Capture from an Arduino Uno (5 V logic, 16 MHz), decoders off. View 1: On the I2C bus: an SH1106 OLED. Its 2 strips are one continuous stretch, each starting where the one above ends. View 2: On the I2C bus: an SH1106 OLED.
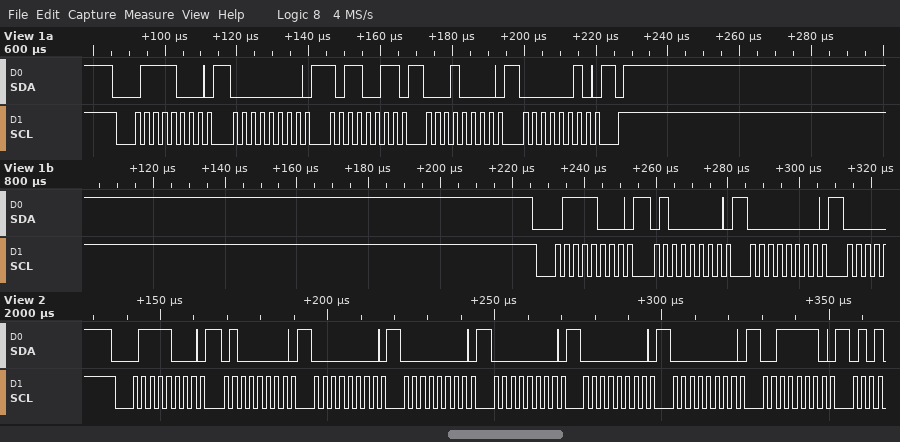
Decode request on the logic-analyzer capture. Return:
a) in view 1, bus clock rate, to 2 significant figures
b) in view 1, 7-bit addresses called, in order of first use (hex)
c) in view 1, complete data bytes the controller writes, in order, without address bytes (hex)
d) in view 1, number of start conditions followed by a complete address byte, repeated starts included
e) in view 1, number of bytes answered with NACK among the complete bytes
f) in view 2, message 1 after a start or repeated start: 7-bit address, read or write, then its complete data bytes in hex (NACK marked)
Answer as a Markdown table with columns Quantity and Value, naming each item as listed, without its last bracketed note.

| Quantity | Value |
|---|---|
| in view 1, bus clock rate, to 2 significant figures | 400 kHz |
| in view 1, 7-bit addresses called, in order of first use | 0x3C |
| in view 1, complete data bytes the controller writes, in order, without address bytes | 00 B3 10 02 40 00 |
| in view 1, number of start conditions followed by a complete address byte, repeated starts included | 2 |
| in view 1, number of bytes answered with NACK among the complete bytes | 0 |
| in view 2, message 1 after a start or repeated start: 7-bit address, read or write, then its complete data bytes in hex | 0x3C write: 40 00 00 00 00 00 3E |
